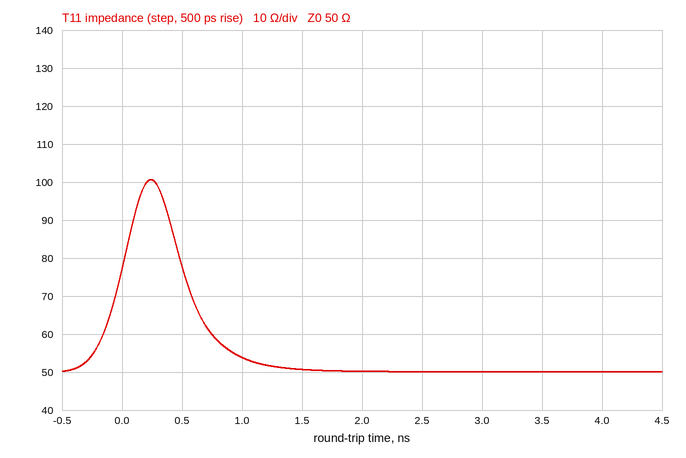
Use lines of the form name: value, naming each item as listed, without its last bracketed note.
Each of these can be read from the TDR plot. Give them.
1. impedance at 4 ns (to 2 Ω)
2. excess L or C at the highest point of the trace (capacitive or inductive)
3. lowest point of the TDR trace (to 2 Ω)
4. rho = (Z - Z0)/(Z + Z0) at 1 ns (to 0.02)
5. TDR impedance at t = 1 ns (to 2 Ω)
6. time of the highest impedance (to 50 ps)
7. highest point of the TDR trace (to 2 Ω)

impedance at 4 ns: 50 Ω
excess L or C at the highest point of the trace: inductive
lowest point of the TDR trace: 50 Ω
rho = (Z - Z0)/(Z + Z0) at 1 ns: +0.04
TDR impedance at t = 1 ns: 54 Ω
time of the highest impedance: 250 ps
highest point of the TDR trace: 100 Ω
